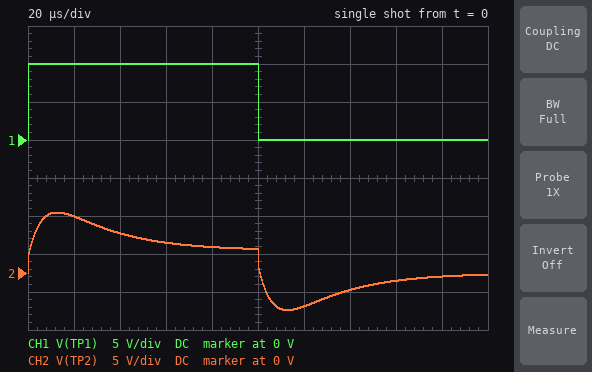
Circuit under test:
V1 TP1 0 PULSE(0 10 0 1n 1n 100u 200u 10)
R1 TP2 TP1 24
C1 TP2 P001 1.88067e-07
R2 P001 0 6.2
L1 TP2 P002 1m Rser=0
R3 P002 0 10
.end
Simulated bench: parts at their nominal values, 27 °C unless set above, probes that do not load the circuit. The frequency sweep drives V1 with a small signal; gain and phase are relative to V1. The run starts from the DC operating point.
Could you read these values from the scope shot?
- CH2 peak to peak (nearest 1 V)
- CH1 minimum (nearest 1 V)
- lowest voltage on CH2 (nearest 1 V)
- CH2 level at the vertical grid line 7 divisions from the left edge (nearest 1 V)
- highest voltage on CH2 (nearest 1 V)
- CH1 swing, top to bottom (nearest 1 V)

13 V
0 V
-5 V
-2 V
8 V
10 V
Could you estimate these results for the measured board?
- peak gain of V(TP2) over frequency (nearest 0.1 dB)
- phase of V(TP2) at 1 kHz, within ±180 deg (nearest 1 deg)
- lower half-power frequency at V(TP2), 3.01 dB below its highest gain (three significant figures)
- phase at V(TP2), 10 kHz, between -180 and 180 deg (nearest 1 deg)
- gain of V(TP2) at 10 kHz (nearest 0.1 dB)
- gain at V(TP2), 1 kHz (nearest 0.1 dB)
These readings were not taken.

-0.6 dB
21 deg
3.97 kHz
5 deg
-0.7 dB
-9.3 dB
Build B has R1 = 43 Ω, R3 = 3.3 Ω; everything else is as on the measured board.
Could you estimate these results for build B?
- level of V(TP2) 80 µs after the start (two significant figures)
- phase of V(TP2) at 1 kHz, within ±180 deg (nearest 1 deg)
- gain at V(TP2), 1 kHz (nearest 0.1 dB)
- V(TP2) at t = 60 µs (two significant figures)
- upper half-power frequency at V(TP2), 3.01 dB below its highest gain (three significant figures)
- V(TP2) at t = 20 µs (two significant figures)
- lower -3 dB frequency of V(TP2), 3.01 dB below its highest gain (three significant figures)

700 mV
54 deg
-16.3 dB
1.2 V
24.2 kHz
6.2 V
5.30 kHz
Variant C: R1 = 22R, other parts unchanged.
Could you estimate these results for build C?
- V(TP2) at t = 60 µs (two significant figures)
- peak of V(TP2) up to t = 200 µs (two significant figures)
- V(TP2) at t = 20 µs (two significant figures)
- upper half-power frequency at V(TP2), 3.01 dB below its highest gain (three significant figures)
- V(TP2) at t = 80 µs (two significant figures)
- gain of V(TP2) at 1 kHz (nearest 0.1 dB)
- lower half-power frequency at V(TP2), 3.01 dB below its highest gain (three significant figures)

4.3 V
8.1 V
7.6 V
38.1 kHz
3.7 V
-8.8 dB
3.75 kHz
